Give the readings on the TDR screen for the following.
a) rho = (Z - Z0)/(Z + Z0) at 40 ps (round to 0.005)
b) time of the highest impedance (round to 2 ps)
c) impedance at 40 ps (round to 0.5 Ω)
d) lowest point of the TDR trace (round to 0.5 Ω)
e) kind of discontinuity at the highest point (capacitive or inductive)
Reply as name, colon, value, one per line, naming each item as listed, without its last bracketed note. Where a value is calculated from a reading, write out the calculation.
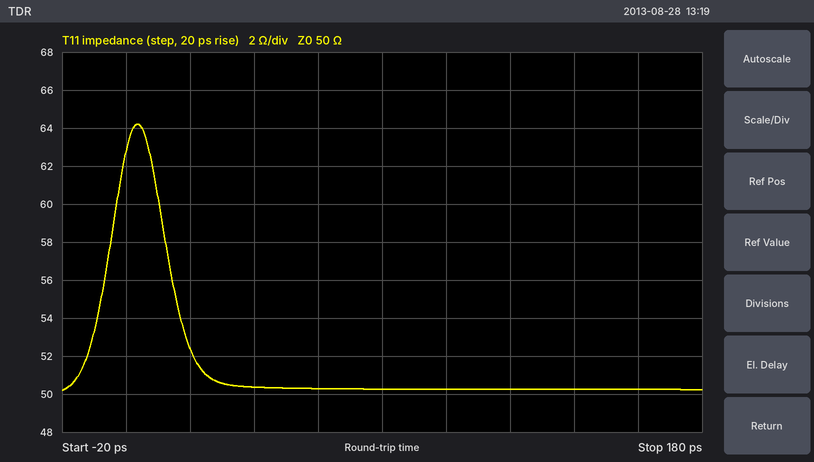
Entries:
rho = (Z - Z0)/(Z + Z0) at 40 ps: (50.5 − 50)/(50.5 + 50) ≈ +0.005
time of the highest impedance: 4 ps
impedance at 40 ps: 50.5 Ω
lowest point of the TDR trace: 50.0 Ω
kind of discontinuity at the highest point: inductive
